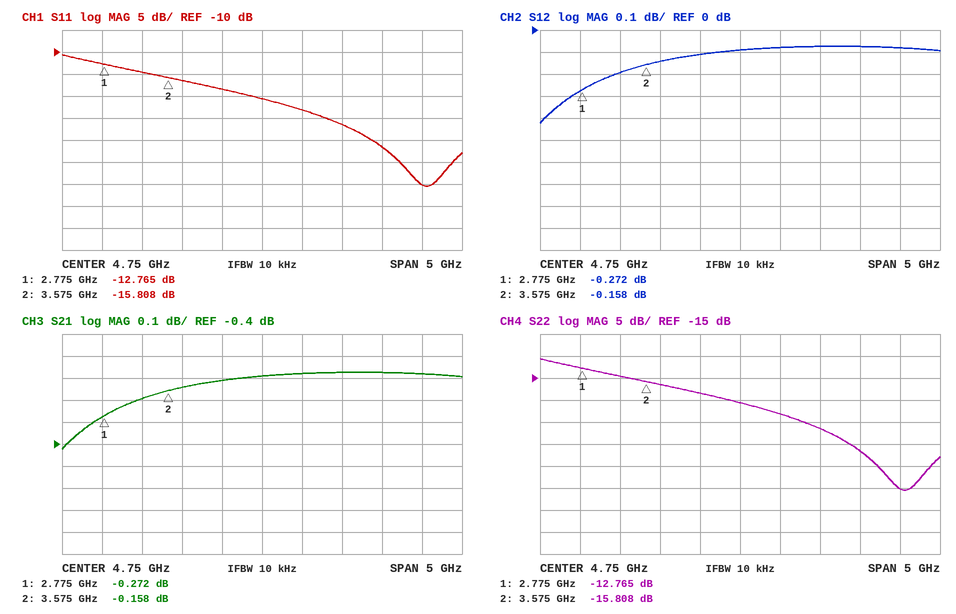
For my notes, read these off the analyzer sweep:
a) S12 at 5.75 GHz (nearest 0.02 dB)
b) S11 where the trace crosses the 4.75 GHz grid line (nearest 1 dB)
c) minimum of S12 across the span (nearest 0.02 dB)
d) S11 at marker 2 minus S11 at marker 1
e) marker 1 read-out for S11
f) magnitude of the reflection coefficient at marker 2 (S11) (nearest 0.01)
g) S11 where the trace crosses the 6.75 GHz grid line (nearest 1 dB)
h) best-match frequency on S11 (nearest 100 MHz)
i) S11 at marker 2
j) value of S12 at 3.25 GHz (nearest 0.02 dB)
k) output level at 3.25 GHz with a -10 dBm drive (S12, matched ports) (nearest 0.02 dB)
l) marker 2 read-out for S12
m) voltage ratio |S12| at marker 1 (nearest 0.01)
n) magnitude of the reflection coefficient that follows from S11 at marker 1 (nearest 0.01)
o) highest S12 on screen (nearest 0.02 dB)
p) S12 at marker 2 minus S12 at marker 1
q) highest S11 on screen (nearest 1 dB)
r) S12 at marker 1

-0.08 dB
-21 dB
-0.42 dB
-3.043 dB
-12.765 dB
0.16
-40 dB
6.8 GHz
-15.808 dB
-0.20 dB
-10.20 dBm
-0.158 dB
0.97
0.23
-0.08 dB
0.114 dB
-11 dB
-0.272 dB
